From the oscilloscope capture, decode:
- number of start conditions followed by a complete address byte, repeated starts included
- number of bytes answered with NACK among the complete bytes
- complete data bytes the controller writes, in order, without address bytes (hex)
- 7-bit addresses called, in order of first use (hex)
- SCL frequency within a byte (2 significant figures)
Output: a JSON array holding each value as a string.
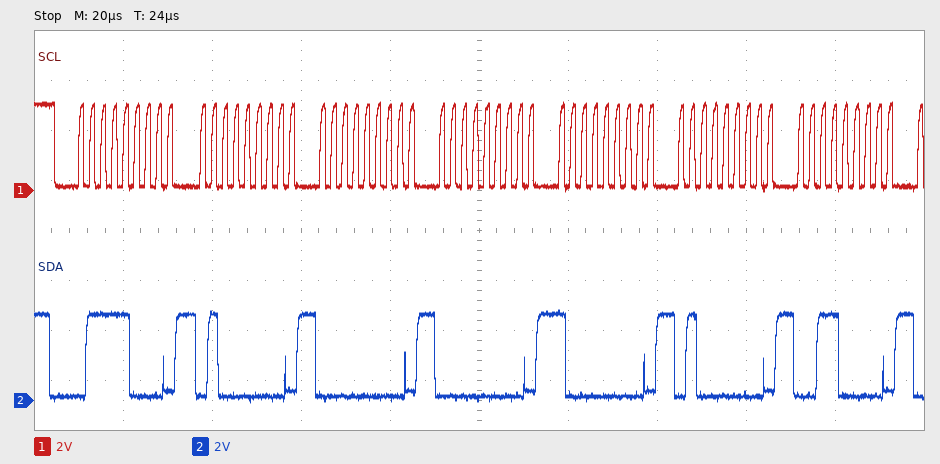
["1", "0", "40 00 00 80 40 30", "0x3C", "400 kHz"]
